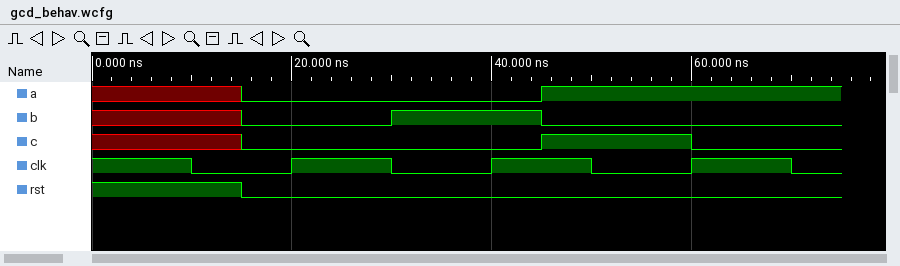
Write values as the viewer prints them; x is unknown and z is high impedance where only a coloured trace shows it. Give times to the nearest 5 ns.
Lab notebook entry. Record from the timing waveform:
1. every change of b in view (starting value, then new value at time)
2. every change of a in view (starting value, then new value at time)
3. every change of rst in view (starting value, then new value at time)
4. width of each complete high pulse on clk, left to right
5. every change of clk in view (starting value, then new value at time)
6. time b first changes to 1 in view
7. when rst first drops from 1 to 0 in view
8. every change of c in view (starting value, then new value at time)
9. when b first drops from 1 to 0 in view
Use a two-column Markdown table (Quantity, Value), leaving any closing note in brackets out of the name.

| Quantity | Value |
|---|---|
| every change of b in view | x, 0 at 15 ns, 1 at 30 ns, 0 at 45 ns |
| every change of a in view | x, 0 at 15 ns, 1 at 45 ns |
| every change of rst in view | 1, 0 at 15 ns |
| width of each complete high pulse on clk, left to right | 10 ns, 10 ns, 10 ns |
| every change of clk in view | 1, 0 at 10 ns, 1 at 20 ns, 0 at 30 ns, 1 at 40 ns, 0 at 50 ns, 1 at 60 ns, 0 at 70 ns |
| time b first changes to 1 in view | 30 ns |
| when rst first drops from 1 to 0 in view | 15 ns |
| every change of c in view | x, 0 at 15 ns, 1 at 45 ns, 0 at 60 ns |
| when b first drops from 1 to 0 in view | 45 ns |
